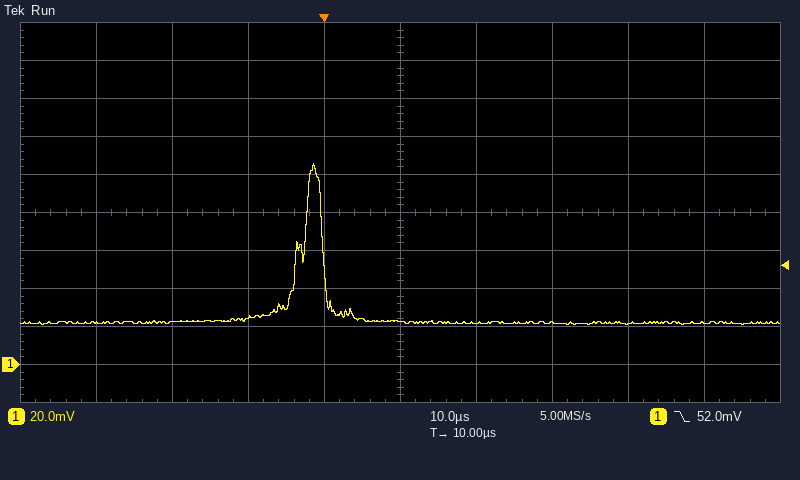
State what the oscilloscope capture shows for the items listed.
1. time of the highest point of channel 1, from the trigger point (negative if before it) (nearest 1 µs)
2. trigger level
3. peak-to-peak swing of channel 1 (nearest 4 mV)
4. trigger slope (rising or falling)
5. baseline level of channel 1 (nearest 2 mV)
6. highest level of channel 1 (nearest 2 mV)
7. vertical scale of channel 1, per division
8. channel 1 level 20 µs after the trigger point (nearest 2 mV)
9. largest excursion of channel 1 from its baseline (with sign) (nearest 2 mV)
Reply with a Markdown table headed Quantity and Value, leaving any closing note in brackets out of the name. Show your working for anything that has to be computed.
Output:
| Quantity | Value |
|---|---|
| time of the highest point of channel 1, from the trigger point (negative if before it) | -1 µs |
| trigger level | 52.0 mV |
| peak-to-peak swing of channel 1 | 84 mV |
| trigger slope | falling |
| baseline level of channel 1 | 22 mV |
| highest level of channel 1 | 106 mV |
| vertical scale of channel 1, per division | 20 mV |
| channel 1 level 20 µs after the trigger point | 22 mV |
| largest excursion of channel 1 from its baseline (with sign) | 106 mV − (22 mV) = +84 mV |
